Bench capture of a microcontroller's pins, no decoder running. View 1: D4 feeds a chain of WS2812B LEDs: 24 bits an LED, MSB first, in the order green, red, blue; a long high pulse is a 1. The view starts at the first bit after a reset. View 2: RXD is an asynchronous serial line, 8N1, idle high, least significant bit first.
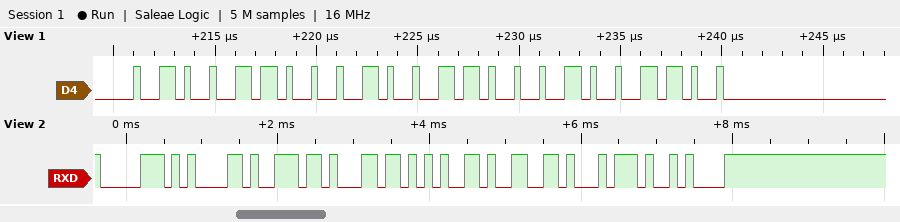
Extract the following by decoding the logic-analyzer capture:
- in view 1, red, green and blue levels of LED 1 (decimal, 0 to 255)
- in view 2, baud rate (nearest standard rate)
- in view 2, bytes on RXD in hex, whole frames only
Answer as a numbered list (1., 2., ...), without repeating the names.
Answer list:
1. 76, 76, 76
2. 9600 baud
3. 70 61 6E 6C 65 66 74 0A
